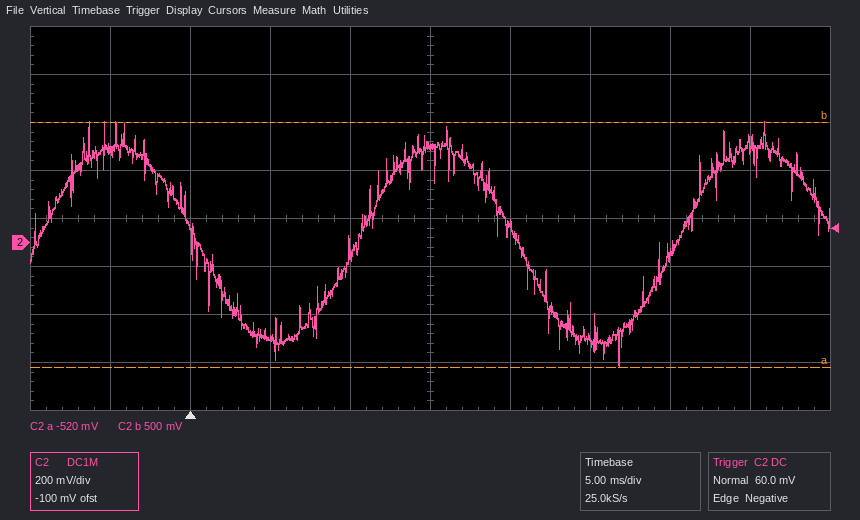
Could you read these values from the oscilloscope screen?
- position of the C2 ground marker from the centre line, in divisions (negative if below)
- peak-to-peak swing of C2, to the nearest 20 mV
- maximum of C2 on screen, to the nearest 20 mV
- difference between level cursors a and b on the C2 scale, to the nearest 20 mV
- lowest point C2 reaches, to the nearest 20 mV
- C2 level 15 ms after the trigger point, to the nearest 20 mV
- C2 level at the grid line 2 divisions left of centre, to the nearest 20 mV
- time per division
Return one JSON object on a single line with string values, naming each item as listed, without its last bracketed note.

{"position of the C2 ground marker from the centre line, in divisions": "-0.5 div", "peak-to-peak swing of C2, to the nearest 20 mV": "1.02 V", "maximum of C2 on screen, to the nearest 20 mV": "500 mV", "difference between level cursors a and b on the C2 scale, to the nearest 20 mV": "1.02 V", "lowest point C2 reaches, to the nearest 20 mV": "-520 mV", "C2 level 15 ms after the trigger point, to the nearest 20 mV": "400 mV", "C2 level at the grid line 2 divisions left of centre, to the nearest 20 mV": "-400 mV", "time per division": "5 ms"}
